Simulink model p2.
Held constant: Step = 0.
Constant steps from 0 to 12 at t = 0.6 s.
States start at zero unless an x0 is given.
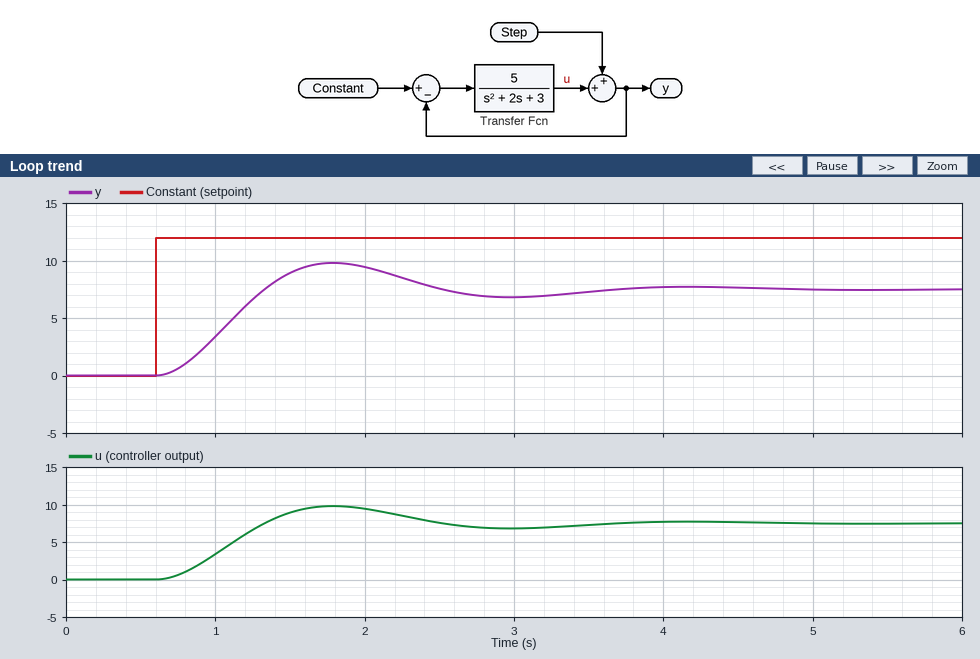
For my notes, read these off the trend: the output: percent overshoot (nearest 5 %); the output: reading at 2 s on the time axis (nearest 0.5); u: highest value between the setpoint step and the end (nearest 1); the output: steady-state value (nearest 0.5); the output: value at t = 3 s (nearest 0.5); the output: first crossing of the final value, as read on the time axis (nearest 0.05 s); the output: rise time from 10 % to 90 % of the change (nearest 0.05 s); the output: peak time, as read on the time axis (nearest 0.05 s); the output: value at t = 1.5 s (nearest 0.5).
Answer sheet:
30 %
9.5
10
7.5
7.0
1.35 s
0.50 s
1.80 s
9.0
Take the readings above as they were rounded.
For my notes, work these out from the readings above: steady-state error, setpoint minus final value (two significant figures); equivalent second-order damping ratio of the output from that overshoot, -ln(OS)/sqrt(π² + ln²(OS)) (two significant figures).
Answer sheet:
4.5
0.36
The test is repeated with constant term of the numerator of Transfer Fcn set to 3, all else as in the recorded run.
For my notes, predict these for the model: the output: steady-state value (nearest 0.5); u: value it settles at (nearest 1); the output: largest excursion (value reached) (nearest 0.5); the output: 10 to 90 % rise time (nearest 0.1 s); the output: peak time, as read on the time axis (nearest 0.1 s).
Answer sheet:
6.0
6
7.5
0.6 s
2.0 s
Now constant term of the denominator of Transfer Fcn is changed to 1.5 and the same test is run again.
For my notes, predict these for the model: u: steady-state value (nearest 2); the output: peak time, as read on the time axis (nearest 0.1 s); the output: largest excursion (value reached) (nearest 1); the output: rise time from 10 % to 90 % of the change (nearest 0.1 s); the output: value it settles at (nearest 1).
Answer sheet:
10
1.9 s
12
0.6 s
9
